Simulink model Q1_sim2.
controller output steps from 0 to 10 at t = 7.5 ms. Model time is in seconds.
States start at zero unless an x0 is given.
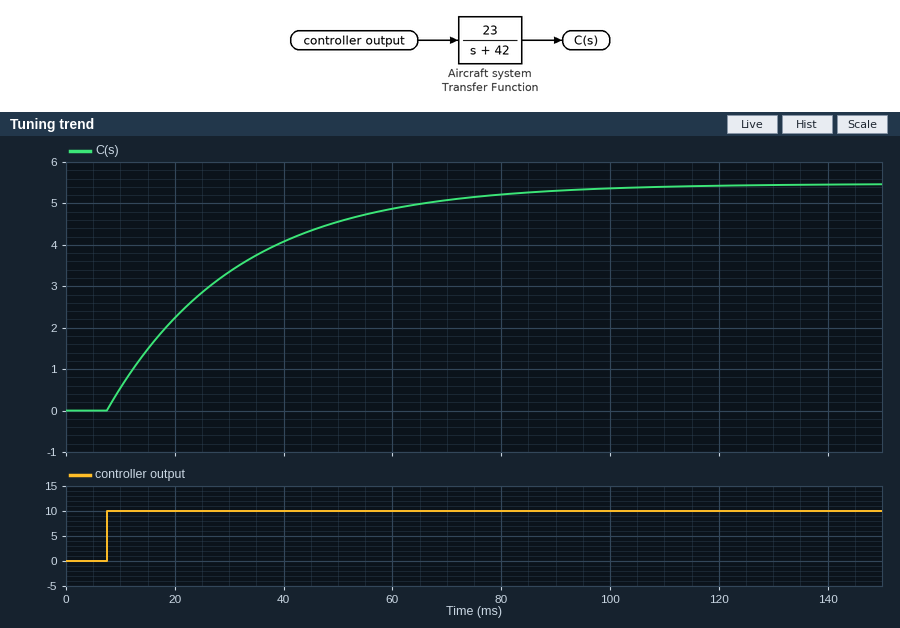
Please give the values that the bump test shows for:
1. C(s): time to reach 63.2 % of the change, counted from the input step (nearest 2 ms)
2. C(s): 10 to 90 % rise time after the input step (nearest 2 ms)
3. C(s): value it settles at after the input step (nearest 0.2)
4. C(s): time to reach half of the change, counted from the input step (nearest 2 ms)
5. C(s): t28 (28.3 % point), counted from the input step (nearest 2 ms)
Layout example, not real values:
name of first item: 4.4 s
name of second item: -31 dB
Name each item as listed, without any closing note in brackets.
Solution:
C(s): time to reach 63.2 % of the change, counted from the input step: 24 ms
C(s): 10 to 90 % rise time after the input step: 52 ms
C(s): value it settles at after the input step: 5.4
C(s): time to reach half of the change, counted from the input step: 16 ms
C(s): t28 (28.3 % point), counted from the input step: 8 ms
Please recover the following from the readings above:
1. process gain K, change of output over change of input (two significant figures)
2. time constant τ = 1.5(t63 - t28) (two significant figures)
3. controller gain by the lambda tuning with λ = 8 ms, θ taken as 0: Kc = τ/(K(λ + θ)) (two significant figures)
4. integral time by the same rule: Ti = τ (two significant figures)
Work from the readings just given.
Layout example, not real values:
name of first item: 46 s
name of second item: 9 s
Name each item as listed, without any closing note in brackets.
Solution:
process gain K, change of output over change of input: 0.54
time constant τ = 1.5(t63 - t28): 24 ms
controller gain by the lambda tuning with λ = 8 ms, θ taken as 0: Kc = τ/(K(λ + θ)): 5.6
integral time by the same rule: Ti = τ: 24 ms
